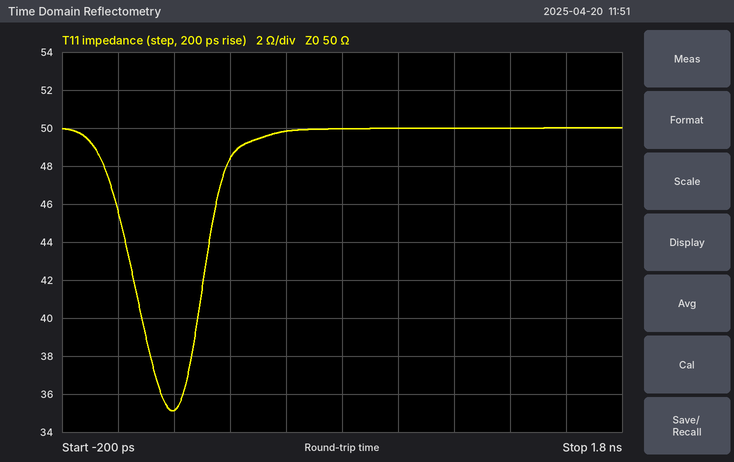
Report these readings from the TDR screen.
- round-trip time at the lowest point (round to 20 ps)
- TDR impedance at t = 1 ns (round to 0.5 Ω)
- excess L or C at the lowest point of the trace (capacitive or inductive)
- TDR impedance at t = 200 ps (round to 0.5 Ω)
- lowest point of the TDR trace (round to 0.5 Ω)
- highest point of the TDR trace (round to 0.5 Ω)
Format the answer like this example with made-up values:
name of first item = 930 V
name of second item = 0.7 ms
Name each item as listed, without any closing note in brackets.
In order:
round-trip time at the lowest point = 200 ps
TDR impedance at t = 1 ns = 50.0 Ω
excess L or C at the lowest point of the trace = capacitive
TDR impedance at t = 200 ps = 35.0 Ω
lowest point of the TDR trace = 35.0 Ω
highest point of the TDR trace = 50.0 Ω
